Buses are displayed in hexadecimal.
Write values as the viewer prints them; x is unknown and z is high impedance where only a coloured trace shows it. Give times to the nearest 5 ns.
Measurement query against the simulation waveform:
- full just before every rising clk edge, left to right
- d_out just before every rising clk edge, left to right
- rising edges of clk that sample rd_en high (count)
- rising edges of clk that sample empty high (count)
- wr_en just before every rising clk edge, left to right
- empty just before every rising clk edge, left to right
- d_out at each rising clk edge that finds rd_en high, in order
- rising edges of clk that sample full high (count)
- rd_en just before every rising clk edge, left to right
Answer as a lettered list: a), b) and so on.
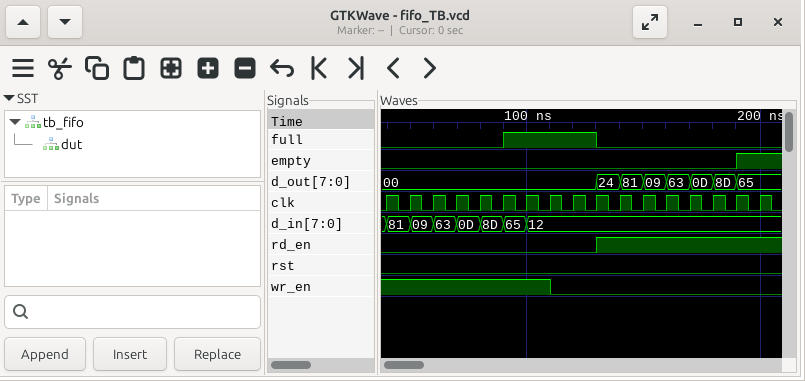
a) 0 0 0 0 0 0 1 1 1 1 0 0 0 0 0 0 0
b) 00, 00, 00, 00, 00, 00, 00, 00, 00, 00, 24, 81, 09, 63, 0D, 8D, 65
c) 7
d) 1
e) 1 1 1 1 1 1 1 1 0 0 0 0 0 0 0 0 0
f) 0 0 0 0 0 0 0 0 0 0 0 0 0 0 0 0 1
g) 24, 81, 09, 63, 0D, 8D, 65
h) 4
i) 0 0 0 0 0 0 0 0 0 0 1 1 1 1 1 1 1
